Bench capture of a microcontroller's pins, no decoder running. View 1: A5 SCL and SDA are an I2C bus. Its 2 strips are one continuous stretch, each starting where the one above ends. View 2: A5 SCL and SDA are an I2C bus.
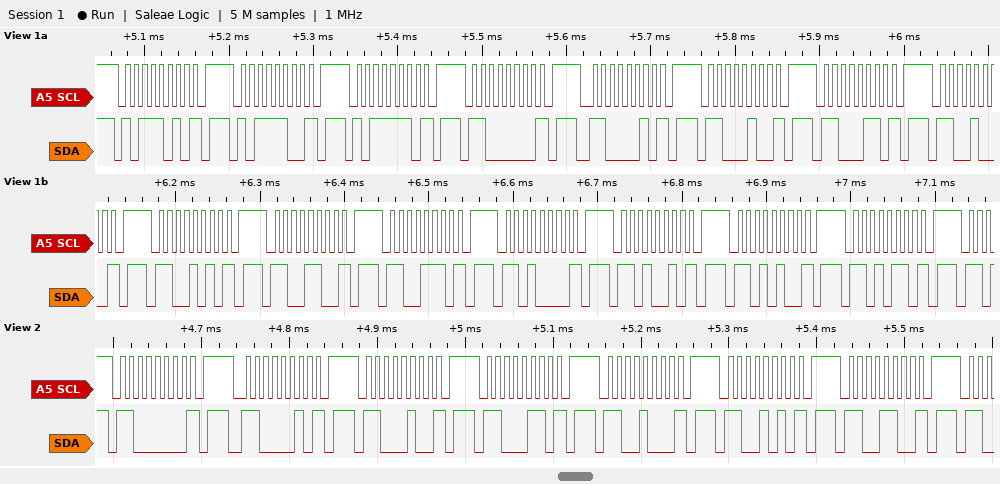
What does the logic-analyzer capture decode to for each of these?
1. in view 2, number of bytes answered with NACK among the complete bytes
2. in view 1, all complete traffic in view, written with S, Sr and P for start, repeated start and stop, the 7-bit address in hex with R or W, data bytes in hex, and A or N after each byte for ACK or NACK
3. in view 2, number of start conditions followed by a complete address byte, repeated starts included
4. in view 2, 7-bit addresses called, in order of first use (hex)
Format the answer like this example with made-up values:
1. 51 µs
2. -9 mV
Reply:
1. 7
2. S 5DW N P S 5EW N P S 5FW N P S 60W N P S 61W N P S 62W N P S 63W N P S 64W N P S 65W N P S 66W N P S 67W N P S 68W N P S 69W N P S 6AW N P S 6BW N P
3. 7
4. 0x60 0x61 0x62 0x63 0x64 0x65 0x66
